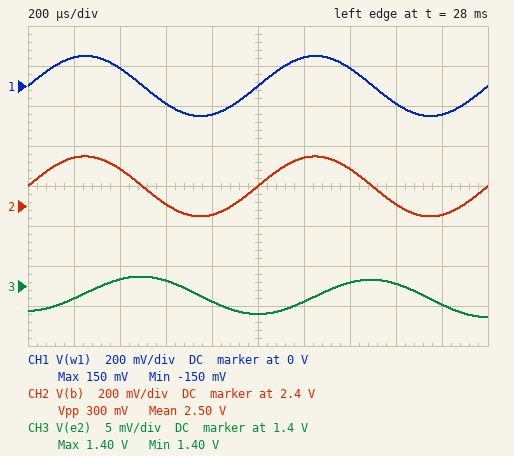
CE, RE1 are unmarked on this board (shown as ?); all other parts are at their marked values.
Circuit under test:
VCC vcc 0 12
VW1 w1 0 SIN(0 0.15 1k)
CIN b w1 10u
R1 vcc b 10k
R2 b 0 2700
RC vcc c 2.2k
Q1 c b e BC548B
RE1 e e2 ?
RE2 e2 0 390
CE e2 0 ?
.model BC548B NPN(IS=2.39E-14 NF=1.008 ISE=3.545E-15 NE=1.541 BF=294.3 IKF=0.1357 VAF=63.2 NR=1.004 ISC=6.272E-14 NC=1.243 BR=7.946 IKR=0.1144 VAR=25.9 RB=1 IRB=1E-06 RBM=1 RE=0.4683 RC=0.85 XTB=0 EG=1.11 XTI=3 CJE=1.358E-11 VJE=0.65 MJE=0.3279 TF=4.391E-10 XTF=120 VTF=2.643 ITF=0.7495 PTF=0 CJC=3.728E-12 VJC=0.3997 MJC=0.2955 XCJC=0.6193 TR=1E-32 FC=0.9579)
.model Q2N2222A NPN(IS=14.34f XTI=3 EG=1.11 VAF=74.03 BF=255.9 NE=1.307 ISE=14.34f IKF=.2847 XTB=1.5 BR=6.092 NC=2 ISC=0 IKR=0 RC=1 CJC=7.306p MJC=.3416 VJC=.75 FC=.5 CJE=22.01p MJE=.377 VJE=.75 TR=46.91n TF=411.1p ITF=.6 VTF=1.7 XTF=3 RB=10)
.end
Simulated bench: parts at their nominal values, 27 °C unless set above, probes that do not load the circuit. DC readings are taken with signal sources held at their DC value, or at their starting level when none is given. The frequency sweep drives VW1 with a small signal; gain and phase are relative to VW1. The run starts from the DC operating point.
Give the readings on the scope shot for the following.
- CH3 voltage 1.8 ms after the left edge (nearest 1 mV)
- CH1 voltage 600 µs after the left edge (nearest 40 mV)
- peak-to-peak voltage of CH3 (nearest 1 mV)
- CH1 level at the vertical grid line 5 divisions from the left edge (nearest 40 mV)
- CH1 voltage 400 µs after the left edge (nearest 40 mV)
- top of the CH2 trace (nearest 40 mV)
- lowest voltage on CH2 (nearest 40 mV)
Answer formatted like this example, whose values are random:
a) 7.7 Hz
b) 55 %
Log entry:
a) 1.398 V
b) -80 mV
c) 5 mV
d) 0 V
e) 80 mV
f) 2.64 V
g) 2.36 V
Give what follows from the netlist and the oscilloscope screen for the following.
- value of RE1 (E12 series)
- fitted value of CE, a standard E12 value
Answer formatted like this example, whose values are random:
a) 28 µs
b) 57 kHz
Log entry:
a) 120 Ω
b) 82 µF
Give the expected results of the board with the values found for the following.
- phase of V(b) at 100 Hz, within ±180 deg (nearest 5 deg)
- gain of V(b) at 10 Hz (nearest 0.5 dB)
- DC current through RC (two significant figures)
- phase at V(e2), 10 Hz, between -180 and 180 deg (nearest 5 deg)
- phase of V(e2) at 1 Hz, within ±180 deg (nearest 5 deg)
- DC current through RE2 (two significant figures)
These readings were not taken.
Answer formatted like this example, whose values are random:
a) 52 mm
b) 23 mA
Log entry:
a) 5 deg
b) -2.0 dB
c) 3.6 mA
d) 10 deg
e) 80 deg
f) 3.6 mA
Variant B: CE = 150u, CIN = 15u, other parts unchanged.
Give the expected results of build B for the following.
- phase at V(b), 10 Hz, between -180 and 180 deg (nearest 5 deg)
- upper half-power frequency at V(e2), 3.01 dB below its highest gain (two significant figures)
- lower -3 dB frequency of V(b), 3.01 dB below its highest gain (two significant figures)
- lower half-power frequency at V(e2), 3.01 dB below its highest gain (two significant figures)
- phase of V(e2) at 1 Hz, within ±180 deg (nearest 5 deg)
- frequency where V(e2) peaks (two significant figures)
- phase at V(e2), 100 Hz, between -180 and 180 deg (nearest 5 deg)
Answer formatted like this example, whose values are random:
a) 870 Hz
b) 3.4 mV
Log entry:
a) 25 deg
b) 19 Hz
c) 5.2 Hz
d) 2.9 Hz
e) 75 deg
f) 7.5 Hz
g) -80 deg
